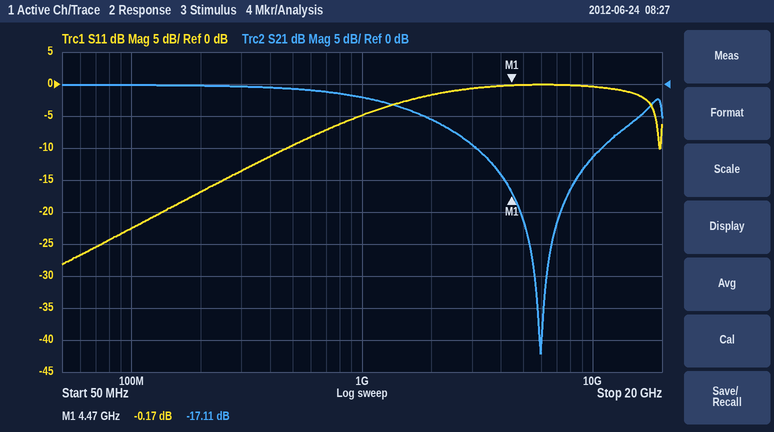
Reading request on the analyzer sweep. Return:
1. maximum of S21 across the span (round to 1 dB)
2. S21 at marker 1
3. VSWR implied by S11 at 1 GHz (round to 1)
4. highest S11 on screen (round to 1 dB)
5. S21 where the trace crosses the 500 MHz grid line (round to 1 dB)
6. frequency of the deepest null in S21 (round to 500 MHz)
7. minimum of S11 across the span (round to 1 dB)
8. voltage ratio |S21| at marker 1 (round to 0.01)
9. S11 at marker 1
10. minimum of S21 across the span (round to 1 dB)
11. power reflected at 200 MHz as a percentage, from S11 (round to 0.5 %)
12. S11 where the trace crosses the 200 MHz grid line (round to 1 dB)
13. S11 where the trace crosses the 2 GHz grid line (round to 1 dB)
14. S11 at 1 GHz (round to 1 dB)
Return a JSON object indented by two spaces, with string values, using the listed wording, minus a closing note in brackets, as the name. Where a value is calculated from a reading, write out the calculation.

{
  "maximum of S21 across the span": "0 dB",
  "S21 at marker 1": "-17.11 dB",
  "VSWR implied by S11 at 1 GHz": "|Γ| = 10^(-5/20) = 0.5623; VSWR = (1 + 0.5623)/(1 − 0.5623) ≈ 4",
  "highest S11 on screen": "0 dB",
  "S21 where the trace crosses the 500 MHz grid line": "-1 dB",
  "frequency of the deepest null in S21": "6.0 GHz",
  "minimum of S11 across the span": "-28 dB",
  "voltage ratio |S21| at marker 1": "10^(-17.11/20) ≈ 0.14",
  "S11 at marker 1": "-0.17 dB",
  "minimum of S21 across the span": "-42 dB",
  "power reflected at 200 MHz as a percentage, from S11": "10^(-17/10) ≈ 2.0 %",
  "S11 where the trace crosses the 200 MHz grid line": "-17 dB",
  "S11 where the trace crosses the 2 GHz grid line": "-2 dB",
  "S11 at 1 GHz": "-5 dB"
}
